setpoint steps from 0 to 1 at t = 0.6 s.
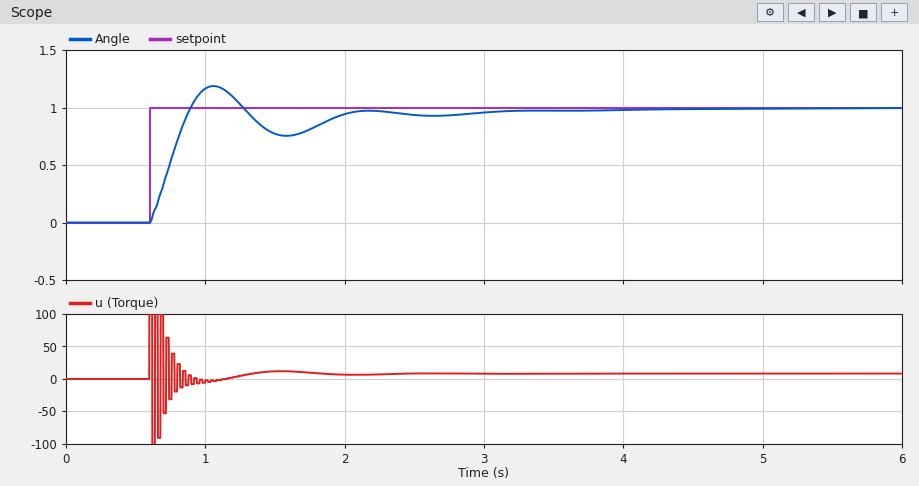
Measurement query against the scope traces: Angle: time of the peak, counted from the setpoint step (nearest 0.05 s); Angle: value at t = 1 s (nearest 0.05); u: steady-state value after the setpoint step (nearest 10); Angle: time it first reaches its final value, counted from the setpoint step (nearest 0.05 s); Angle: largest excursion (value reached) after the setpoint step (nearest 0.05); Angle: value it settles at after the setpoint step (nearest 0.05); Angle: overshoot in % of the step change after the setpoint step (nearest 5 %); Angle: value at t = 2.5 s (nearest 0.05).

0.45 s
1.15
10
0.30 s
1.20
1.00
20 %
0.95
